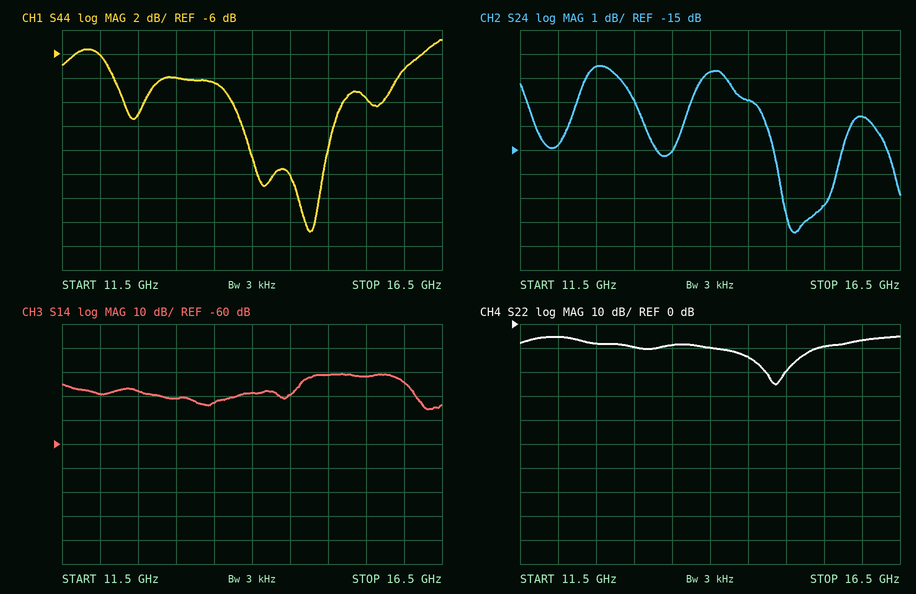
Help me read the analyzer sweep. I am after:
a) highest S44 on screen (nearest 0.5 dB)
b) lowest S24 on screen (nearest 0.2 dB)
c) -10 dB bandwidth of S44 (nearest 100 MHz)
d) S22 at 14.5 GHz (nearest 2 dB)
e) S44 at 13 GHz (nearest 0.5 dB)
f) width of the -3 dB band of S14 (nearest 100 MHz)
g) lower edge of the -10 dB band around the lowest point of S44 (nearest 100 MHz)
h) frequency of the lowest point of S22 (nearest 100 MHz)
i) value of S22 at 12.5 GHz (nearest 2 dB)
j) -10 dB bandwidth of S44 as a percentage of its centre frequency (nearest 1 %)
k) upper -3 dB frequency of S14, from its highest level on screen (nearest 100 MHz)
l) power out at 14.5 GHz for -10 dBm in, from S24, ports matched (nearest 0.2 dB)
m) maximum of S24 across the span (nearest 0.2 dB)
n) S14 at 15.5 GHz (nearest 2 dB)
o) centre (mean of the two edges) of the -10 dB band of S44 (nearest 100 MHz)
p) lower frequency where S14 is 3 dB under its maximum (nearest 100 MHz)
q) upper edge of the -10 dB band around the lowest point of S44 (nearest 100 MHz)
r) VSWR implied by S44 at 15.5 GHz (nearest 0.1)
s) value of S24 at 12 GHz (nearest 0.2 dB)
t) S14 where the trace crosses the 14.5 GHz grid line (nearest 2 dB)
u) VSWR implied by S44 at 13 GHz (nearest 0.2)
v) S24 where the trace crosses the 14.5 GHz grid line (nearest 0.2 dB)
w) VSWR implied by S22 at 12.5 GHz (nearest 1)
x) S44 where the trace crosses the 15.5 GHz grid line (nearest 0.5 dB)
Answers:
-5.0 dB
-18.4 dB
1.5 GHz
-14 dB
-8.0 dB
1.3 GHz
13.7 GHz
14.9 GHz
-8 dB
10 %
16.0 GHz
-23.0 dBm
-11.4 dB
-32 dB
14.5 GHz
14.7 GHz
15.2 GHz
2.0
-14.8 dB
-40 dB
2.4
-13.0 dB
2
-9.5 dB
